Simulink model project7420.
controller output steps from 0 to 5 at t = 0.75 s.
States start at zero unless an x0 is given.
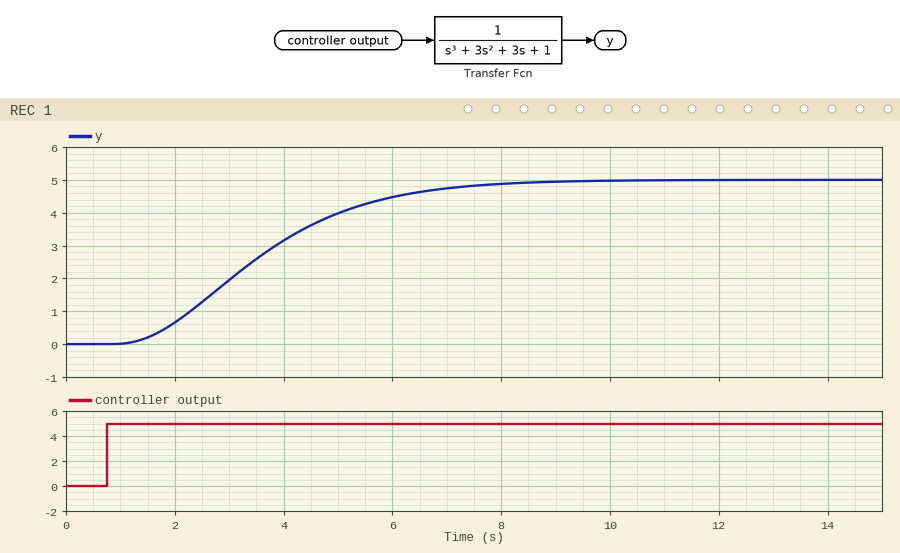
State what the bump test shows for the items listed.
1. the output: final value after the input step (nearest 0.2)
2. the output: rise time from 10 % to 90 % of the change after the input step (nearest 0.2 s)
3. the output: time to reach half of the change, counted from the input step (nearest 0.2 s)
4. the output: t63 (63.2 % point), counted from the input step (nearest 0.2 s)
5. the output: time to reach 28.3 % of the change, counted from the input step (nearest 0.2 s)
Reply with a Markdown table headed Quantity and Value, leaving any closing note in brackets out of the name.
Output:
| Quantity | Value |
|---|---|
| the output: final value after the input step | 5.0 |
| the output: rise time from 10 % to 90 % of the change after the input step | 4.2 s |
| the output: time to reach half of the change, counted from the input step | 2.6 s |
| the output: t63 (63.2 % point), counted from the input step | 3.2 s |
| the output: time to reach 28.3 % of the change, counted from the input step | 1.8 s |
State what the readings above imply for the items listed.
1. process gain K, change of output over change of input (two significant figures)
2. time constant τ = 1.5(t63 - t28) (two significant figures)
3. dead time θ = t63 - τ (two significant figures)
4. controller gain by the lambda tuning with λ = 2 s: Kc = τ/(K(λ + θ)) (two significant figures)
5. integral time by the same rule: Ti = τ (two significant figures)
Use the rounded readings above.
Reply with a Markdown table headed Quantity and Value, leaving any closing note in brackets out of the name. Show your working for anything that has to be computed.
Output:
| Quantity | Value |
|---|---|
| process gain K, change of output over change of input | (5 - 0) / 5 = 1.0 |
| time constant τ = 1.5(t63 - t28) | 1.5 × (3.2 - 1.8) = 2.1 s |
| dead time θ = t63 - τ | 3.2 - 2.1 = 1.1 s |
| controller gain by the lambda tuning with λ = 2 s: Kc = τ/(K(λ + θ)) | 2.1 / (1 × (2 + 1.1)) = 0.68 |
| integral time by the same rule: Ti = τ | 2.1 s |
